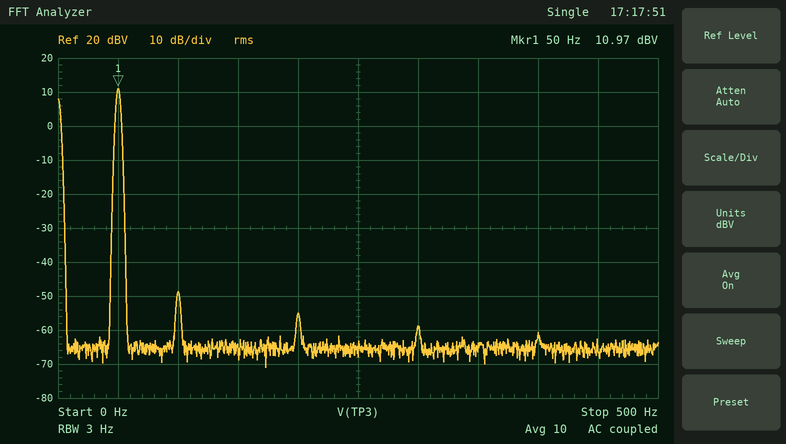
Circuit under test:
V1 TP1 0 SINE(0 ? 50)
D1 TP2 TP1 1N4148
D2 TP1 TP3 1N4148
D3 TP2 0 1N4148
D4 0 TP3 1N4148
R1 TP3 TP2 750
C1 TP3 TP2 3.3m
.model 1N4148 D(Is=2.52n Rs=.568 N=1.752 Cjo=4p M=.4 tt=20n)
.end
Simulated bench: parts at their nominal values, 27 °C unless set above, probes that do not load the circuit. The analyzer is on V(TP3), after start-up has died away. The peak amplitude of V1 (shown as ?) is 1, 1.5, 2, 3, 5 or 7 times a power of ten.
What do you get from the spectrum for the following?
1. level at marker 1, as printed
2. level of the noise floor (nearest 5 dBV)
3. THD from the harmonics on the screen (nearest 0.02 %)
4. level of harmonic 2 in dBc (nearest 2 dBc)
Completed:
10.97 dBV
-65 dBV
0.10 %
-60 dBc
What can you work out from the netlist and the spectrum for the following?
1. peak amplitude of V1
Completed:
10 V
